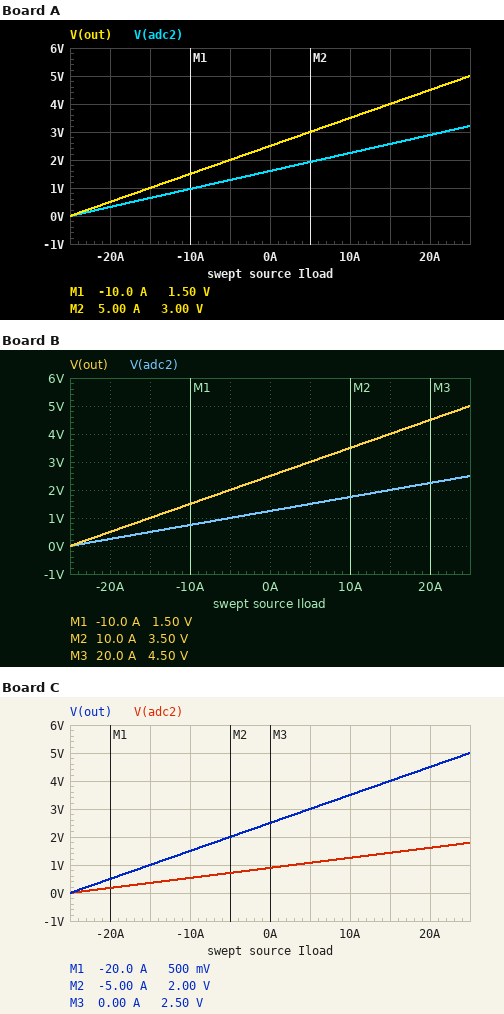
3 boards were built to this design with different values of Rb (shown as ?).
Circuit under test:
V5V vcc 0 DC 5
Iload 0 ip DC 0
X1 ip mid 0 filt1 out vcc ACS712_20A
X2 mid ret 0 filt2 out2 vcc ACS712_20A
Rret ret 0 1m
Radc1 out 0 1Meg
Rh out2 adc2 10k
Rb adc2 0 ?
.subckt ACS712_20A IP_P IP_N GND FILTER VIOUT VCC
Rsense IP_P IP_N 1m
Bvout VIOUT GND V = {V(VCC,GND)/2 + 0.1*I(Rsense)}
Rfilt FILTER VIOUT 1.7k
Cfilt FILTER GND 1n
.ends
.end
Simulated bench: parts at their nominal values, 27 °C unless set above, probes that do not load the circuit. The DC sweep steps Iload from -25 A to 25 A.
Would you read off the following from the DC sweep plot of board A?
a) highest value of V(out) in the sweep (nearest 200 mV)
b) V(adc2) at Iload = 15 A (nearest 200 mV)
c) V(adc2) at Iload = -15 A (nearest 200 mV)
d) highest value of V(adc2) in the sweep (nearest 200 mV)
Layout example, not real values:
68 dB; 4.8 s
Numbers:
5.0 V; 2.6 V; 600 mV; 3.2 V
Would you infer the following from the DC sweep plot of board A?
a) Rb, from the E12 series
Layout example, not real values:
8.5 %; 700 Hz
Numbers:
18 kΩ
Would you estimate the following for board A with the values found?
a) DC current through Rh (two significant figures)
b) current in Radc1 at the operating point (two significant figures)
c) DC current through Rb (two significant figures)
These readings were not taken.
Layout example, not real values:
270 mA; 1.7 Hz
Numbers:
89 µA; 2.5 µA; 89 µA
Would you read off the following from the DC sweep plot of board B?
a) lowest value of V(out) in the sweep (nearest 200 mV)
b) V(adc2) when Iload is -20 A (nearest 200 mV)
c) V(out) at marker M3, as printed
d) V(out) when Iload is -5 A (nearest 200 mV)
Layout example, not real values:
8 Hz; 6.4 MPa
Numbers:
0 V; 200 mV; 4.50 V; 2.0 V
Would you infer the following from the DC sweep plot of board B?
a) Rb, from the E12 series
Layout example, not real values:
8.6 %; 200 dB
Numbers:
10 kΩ
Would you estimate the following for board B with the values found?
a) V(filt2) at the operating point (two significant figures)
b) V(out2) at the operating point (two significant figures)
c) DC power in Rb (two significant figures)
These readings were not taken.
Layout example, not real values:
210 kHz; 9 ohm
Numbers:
2.5 V; 2.5 V; 160 µW
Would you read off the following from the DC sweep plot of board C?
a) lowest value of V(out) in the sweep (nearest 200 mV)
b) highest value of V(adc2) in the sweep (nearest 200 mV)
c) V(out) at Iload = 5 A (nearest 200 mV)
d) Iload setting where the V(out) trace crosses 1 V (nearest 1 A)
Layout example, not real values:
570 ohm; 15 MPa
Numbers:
0 V; 1.8 V; 3.0 V; -15 A
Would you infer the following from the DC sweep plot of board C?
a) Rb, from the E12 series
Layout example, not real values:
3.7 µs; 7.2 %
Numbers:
5.6 kΩ
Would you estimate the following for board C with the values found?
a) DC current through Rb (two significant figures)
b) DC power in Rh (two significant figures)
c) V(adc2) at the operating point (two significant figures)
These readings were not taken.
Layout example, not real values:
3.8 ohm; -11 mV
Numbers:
160 µA; 260 µW; 900 mV
